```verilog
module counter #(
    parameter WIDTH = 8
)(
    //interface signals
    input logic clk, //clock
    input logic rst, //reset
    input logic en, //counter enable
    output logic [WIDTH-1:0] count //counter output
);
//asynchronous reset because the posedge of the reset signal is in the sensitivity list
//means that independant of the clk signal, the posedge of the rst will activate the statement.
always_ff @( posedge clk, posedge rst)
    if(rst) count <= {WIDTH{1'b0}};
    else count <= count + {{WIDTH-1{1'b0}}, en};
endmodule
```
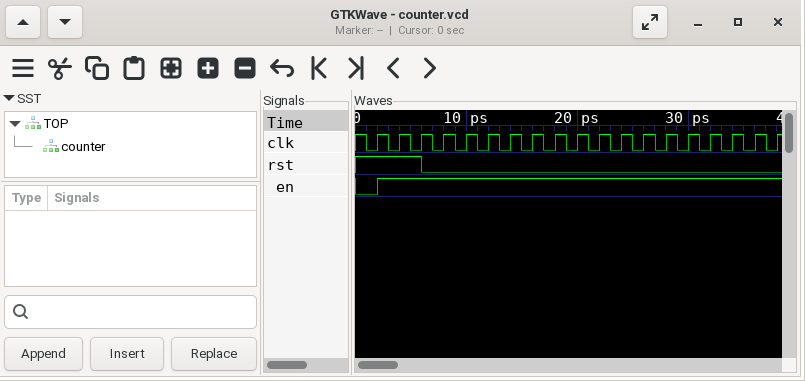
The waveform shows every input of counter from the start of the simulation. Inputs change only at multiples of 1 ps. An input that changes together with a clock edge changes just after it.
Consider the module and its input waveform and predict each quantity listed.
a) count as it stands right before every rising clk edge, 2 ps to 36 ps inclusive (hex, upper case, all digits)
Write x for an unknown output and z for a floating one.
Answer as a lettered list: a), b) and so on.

a) 00, 00, 00, 00, 01, 02, 03, 04, 05, 06, 07, 08, 09, 0A, 0B, 0C, 0D, 0E
